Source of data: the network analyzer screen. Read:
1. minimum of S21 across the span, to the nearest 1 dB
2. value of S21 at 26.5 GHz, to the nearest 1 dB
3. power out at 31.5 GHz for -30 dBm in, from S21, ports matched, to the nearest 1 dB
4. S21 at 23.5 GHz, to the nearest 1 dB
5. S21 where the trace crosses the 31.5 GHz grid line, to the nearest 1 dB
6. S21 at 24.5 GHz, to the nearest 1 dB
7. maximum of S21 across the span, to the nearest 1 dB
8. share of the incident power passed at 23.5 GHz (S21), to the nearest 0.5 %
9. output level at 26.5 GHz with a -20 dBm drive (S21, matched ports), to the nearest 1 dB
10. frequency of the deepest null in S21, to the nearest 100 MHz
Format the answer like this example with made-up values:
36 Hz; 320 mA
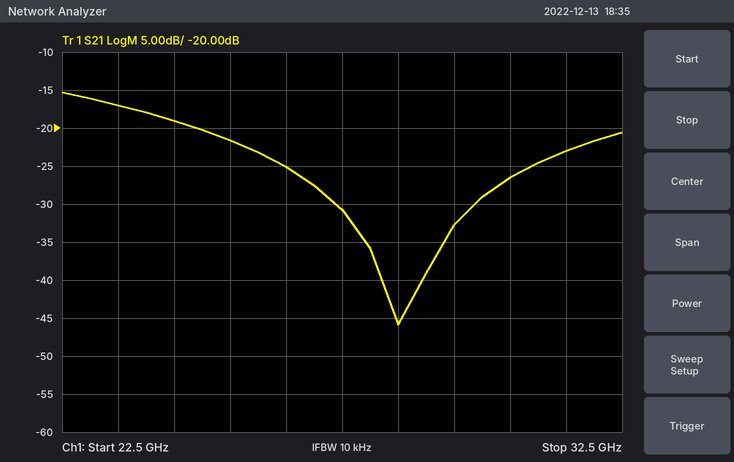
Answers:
-46 dB; -25 dB; -53 dBm; -17 dB; -23 dB; -19 dB; -15 dB; 2.0 %; -45 dBm; 28.5 GHz
